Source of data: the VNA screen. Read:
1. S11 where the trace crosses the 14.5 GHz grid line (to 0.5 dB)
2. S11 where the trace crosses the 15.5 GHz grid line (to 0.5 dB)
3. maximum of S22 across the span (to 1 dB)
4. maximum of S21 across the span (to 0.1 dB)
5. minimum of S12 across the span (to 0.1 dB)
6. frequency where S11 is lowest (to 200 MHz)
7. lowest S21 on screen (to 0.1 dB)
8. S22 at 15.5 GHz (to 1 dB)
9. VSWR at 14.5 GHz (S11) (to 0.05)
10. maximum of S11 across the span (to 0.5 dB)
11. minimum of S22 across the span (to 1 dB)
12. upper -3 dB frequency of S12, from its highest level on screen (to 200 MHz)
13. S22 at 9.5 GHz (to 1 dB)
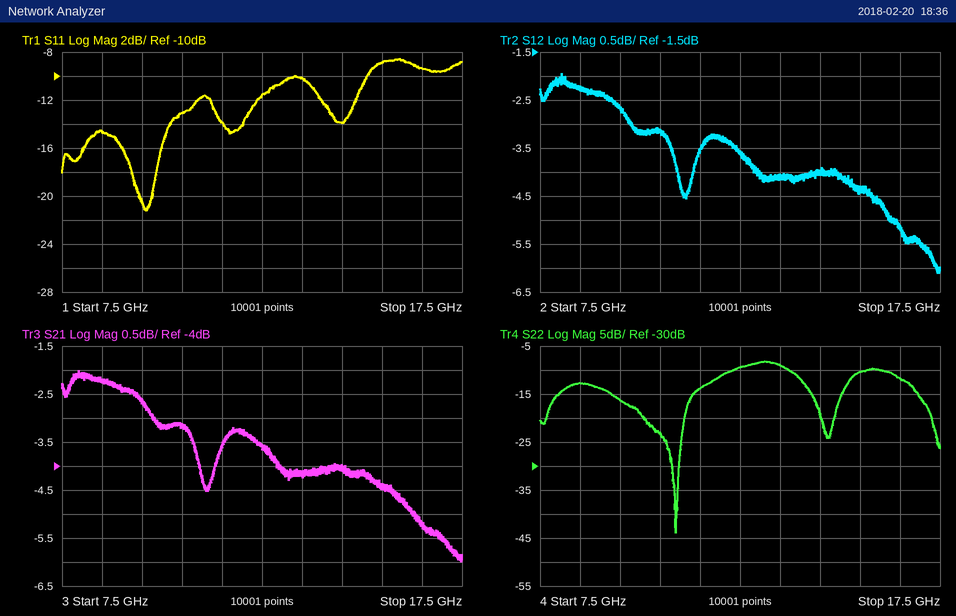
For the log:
-14.0 dB
-9.0 dB
-8 dB
-2.0 dB
-6.1 dB
9.6 GHz
-6.0 dB
-10 dB
1.50
-8.5 dB
-44 dB
16.2 GHz
-16 dB
